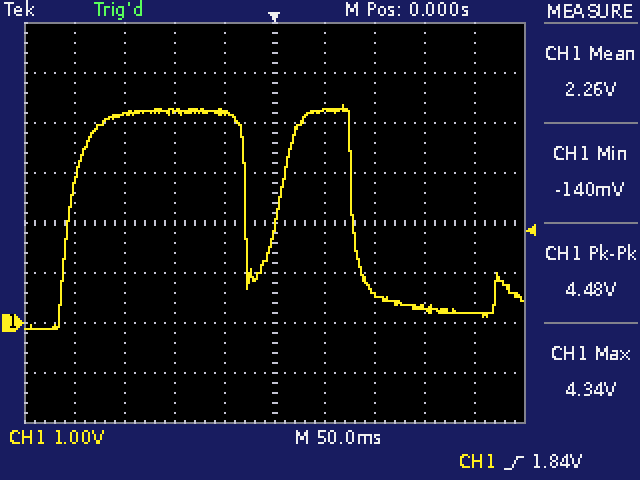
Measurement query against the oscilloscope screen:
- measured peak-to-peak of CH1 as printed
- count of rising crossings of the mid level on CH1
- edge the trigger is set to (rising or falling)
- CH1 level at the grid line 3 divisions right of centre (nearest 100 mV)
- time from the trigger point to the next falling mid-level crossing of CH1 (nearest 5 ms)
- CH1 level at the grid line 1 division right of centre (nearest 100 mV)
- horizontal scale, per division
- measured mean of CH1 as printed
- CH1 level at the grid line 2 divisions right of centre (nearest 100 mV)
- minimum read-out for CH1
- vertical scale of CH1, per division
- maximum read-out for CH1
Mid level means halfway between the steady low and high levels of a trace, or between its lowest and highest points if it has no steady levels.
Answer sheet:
4.48 V
2
rising
300 mV
80 ms
4.3 V
50 ms
2.26 V
600 mV
-140 mV
1 V
4.34 V
